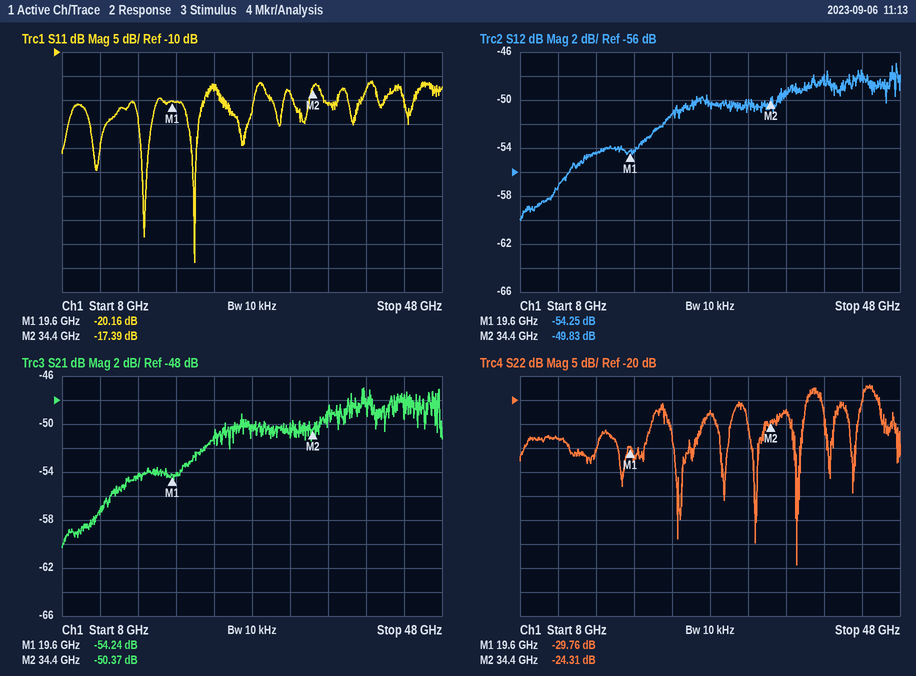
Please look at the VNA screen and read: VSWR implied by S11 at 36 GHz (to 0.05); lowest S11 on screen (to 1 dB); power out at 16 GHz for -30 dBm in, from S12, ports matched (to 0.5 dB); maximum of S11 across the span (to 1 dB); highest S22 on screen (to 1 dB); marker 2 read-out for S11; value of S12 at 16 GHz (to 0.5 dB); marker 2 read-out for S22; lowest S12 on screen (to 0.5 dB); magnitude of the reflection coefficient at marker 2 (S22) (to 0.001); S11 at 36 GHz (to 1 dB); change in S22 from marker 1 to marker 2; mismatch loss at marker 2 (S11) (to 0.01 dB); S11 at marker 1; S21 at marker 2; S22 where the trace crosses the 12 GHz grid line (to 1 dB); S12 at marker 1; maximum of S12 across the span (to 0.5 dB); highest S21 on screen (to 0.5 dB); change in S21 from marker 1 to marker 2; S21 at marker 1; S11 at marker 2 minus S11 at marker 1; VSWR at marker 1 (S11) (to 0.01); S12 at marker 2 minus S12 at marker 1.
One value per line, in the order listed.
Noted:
1.20
-54 dB
-84.5 dBm
-16 dB
-17 dB
-17.39 dB
-54.5 dB
-24.31 dB
-60.0 dB
0.061
-21 dB
5.45 dB
0.08 dB
-20.16 dB
-50.37 dB
-28 dB
-54.25 dB
-47.0 dB
-47.0 dB
3.87 dB
-54.24 dB
2.77 dB
1.22
4.42 dB
